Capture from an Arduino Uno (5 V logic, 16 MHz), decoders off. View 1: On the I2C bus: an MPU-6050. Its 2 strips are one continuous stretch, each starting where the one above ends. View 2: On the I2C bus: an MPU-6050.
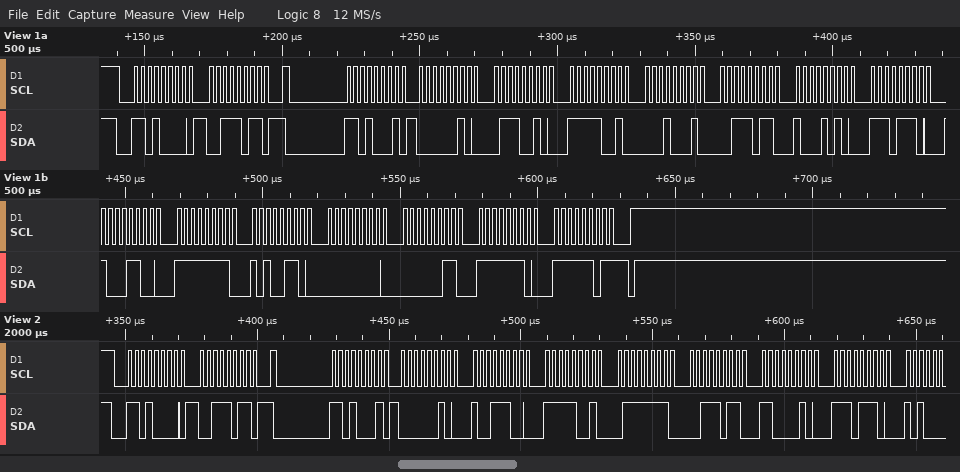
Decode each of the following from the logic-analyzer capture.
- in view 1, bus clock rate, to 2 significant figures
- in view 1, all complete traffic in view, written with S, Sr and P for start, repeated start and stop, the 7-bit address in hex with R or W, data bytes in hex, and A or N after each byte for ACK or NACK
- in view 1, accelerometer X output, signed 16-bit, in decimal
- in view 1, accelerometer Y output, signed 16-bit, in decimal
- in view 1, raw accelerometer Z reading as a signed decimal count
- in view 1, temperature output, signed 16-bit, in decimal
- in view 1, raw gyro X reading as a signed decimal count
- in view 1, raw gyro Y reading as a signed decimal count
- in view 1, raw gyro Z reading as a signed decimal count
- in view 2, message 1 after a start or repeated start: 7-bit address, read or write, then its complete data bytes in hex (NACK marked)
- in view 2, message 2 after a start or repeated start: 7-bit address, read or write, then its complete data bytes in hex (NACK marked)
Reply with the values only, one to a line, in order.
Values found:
400 kHz
S 68W A 3B A Sr 68R A 02 A 72 A F9 A 11 A 3B A 8A A EE A 8C A FF A A6 A 00 A 03 A FE A FD N P
626
-1775
15242
-4468
-90
3
-259
0x68 write: 3B
0x68 read: 02 9C F9 7F 3B C2 EE
